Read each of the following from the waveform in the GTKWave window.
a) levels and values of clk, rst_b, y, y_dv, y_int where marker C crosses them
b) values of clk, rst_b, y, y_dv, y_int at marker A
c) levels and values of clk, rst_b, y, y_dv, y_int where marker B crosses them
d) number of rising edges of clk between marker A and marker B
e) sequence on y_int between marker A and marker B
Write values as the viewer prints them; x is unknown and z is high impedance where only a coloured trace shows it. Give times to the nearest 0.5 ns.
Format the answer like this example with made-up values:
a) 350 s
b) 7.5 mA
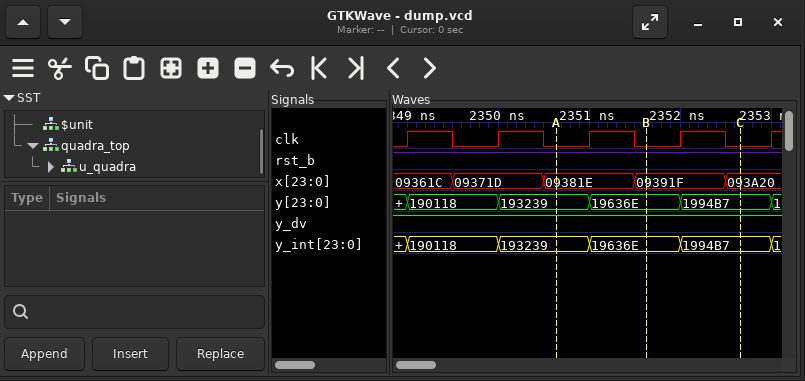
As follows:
a) clk=0, rst_b=1, y=1994B7, y_dv=1, y_int=1994B7
b) clk=0, rst_b=1, y=193239, y_dv=1, y_int=193239
c) clk=0, rst_b=1, y=19636E, y_dv=1, y_int=19636E
d) 1
e) 193239, 19636E
